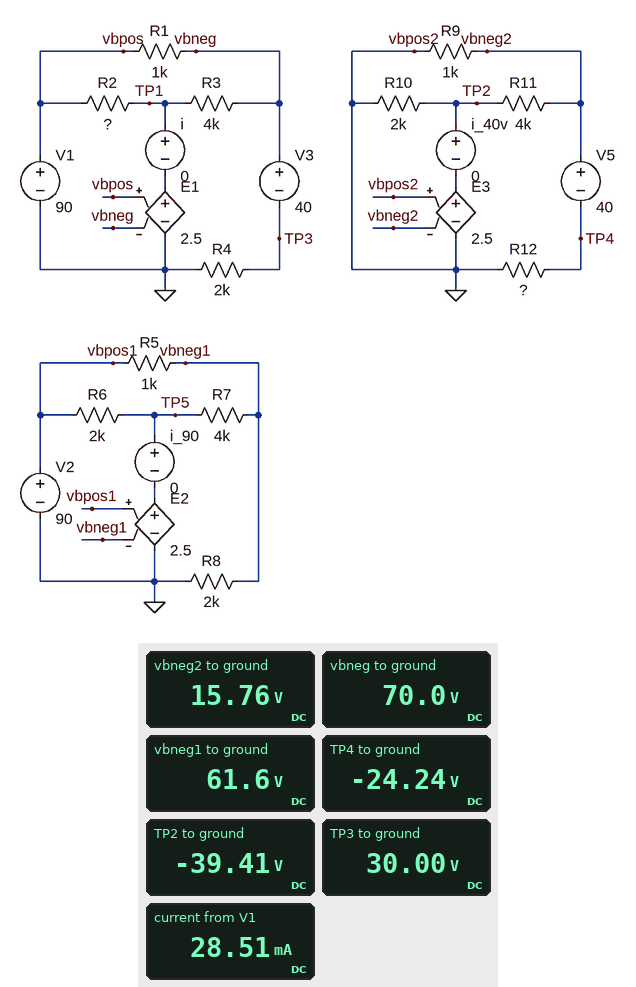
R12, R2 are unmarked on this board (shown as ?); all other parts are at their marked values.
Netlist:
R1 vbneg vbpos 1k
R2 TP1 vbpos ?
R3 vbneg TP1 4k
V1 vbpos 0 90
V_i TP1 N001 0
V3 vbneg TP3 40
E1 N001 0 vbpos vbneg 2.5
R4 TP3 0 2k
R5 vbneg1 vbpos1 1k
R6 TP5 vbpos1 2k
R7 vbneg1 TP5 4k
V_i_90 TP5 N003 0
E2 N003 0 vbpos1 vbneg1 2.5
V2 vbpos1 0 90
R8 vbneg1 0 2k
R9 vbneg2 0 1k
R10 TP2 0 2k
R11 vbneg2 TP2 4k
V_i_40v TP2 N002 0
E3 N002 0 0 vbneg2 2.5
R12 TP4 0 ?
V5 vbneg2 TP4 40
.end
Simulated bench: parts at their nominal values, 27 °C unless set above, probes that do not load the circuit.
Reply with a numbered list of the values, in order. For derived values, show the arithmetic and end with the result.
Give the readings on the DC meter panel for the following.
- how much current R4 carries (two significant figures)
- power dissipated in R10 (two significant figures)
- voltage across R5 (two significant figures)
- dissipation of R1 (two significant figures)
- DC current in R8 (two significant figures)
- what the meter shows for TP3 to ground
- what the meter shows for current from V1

1. (30 V) / 2 kΩ = 15 mA
2. (0 V - (-39.41 V))^2 / 2 kΩ = 780 mW
3. 90 V - 61.6 V = 28 V
4. (90 V - 70 V)^2 / 1 kΩ = 400 mW
5. (61.6 V) / 2 kΩ = 31 mA
6. 30.00 V
7. 28.51 mA
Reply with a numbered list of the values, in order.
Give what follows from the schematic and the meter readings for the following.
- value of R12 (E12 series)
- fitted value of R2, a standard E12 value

1. 820 Ω
2. 4.7 kΩ
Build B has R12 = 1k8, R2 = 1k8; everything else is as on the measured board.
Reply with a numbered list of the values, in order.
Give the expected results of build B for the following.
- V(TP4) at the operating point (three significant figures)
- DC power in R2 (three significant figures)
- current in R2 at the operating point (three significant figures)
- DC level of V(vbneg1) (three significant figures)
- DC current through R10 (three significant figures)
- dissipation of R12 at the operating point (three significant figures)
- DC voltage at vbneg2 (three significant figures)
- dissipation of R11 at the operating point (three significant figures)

1. -30.9 V
2. 889 mW
3. 22.2 mA
4. 61.6 V
5. 11.4 mA
6. 529 mW
7. 9.14 V
8. 256 mW
